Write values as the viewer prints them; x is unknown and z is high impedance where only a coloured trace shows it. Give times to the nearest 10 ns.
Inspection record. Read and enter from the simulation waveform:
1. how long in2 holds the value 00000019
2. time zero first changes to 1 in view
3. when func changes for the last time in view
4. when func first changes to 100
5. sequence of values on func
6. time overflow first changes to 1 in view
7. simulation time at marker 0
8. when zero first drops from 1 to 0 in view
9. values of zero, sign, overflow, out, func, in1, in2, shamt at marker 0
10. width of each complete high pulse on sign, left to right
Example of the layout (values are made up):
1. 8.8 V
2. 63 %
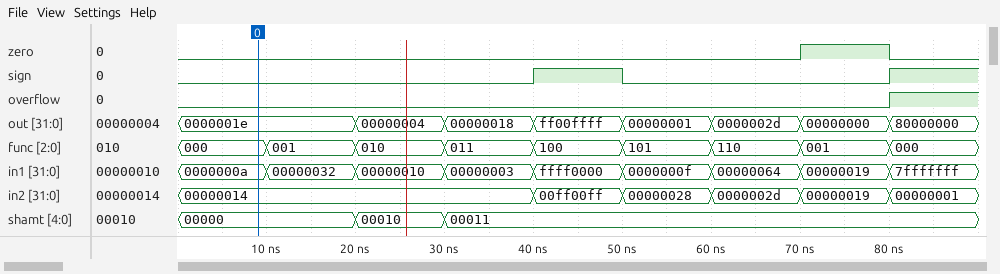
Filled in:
1. 10 ns
2. 70 ns
3. 80 ns
4. 40 ns
5. 000, 001, 010, 011, 100, 101, 110, 001, 000
6. 80 ns
7. 10 ns
8. 80 ns
9. zero=0, sign=0, overflow=0, out=0000001e, func=000, in1=0000000a, in2=00000014, shamt=00000
10. 10 ns
